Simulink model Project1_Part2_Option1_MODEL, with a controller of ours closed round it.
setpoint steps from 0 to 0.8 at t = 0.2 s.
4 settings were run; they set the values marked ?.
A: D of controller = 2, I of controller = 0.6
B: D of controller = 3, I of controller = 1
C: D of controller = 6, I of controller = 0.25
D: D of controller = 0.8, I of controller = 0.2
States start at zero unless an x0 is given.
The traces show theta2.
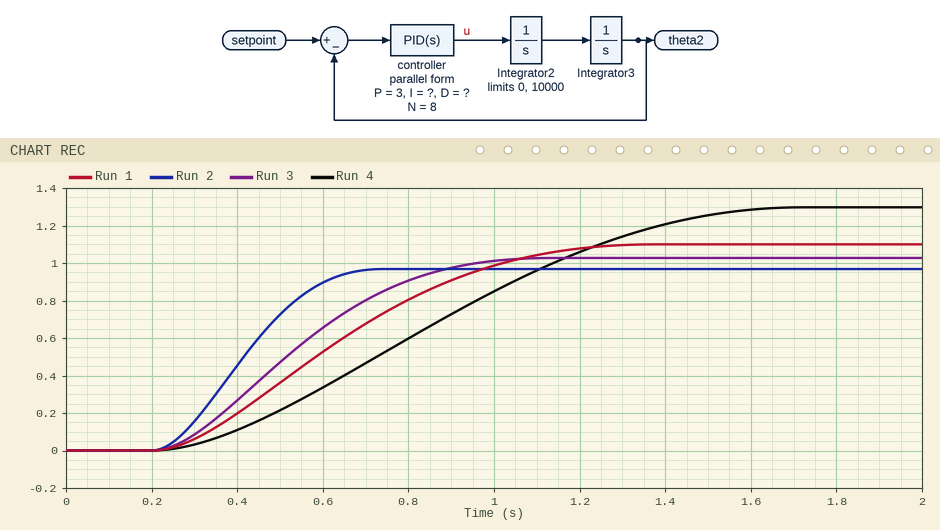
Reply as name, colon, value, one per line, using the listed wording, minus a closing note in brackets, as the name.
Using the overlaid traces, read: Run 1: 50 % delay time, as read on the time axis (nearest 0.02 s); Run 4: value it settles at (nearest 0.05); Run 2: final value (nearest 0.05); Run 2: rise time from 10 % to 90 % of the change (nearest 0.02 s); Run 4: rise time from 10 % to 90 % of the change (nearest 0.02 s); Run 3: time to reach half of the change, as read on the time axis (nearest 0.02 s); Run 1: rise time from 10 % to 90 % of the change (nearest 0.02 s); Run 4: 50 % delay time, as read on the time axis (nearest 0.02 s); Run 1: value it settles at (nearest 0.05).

Run 1: 50 % delay time, as read on the time axis: 0.62 s
Run 4: value it settles at: 1.30
Run 2: final value: 0.95
Run 2: rise time from 10 % to 90 % of the change: 0.30 s
Run 4: rise time from 10 % to 90 % of the change: 0.92 s
Run 3: time to reach half of the change, as read on the time axis: 0.52 s
Run 1: rise time from 10 % to 90 % of the change: 0.66 s
Run 4: 50 % delay time, as read on the time axis: 0.84 s
Run 1: value it settles at: 1.10
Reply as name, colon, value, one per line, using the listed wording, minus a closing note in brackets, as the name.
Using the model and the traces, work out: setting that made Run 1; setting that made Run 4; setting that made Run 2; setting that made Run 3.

setting that made Run 1: A
setting that made Run 4: D
setting that made Run 2: C
setting that made Run 3: B
